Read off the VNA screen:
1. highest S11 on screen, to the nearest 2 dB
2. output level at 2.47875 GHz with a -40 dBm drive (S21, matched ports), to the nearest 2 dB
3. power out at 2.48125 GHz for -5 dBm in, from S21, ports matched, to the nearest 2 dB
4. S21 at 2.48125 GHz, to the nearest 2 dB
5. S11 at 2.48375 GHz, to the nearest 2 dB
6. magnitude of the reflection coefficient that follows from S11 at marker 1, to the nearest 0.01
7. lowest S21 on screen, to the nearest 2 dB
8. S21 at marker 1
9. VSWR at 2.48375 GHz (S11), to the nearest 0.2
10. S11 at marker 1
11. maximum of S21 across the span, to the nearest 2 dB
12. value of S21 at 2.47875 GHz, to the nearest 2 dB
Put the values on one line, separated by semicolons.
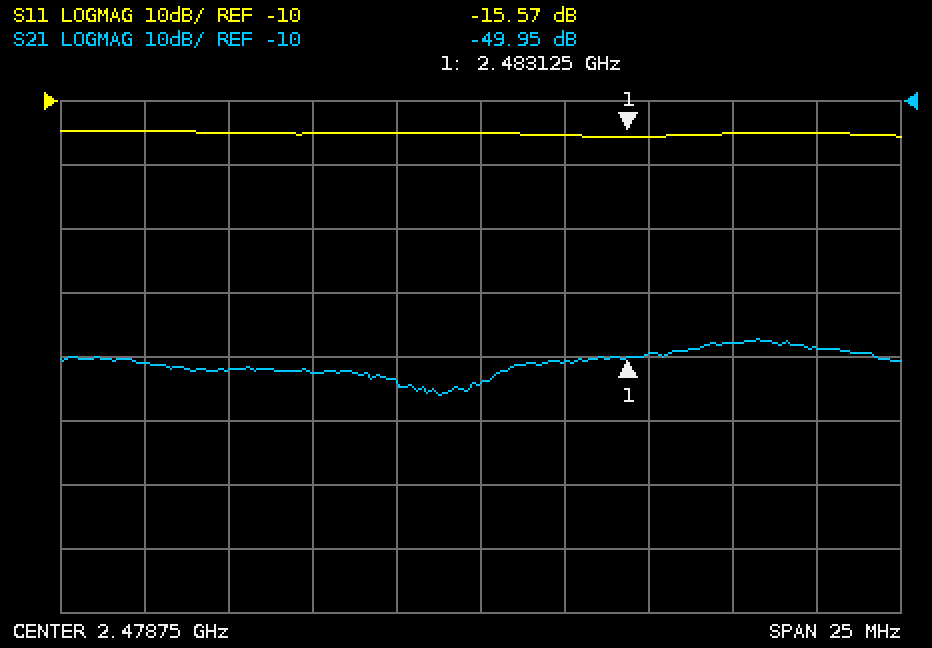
-14 dB; -94 dBm; -56 dBm; -50 dB; -16 dB; 0.17; -56 dB; -49.95 dB; 1.4; -15.57 dB; -48 dB; -54 dB
